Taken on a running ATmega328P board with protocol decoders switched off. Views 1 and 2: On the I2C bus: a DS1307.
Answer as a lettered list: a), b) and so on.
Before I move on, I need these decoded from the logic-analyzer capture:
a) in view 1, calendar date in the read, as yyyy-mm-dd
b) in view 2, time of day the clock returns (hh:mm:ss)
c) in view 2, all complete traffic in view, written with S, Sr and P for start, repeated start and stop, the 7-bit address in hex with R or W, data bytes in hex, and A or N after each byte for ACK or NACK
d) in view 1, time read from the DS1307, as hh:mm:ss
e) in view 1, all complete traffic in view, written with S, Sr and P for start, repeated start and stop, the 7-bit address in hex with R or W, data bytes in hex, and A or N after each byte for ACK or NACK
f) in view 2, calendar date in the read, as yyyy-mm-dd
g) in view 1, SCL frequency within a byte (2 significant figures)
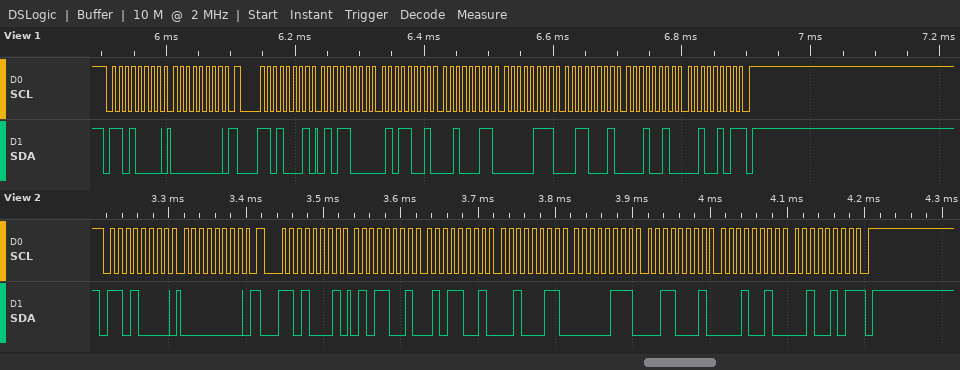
a) 2025-12-31
b) 23:59:59
c) S 68W A 00 A Sr 68R A 59 A 59 A 23 A 07 A 31 A 12 A 25 N P
d) 23:59:58
e) S 68W A 00 A Sr 68R A 58 A 59 A 23 A 07 A 31 A 12 A 25 N P
f) 2025-12-31
g) 100 kHz
